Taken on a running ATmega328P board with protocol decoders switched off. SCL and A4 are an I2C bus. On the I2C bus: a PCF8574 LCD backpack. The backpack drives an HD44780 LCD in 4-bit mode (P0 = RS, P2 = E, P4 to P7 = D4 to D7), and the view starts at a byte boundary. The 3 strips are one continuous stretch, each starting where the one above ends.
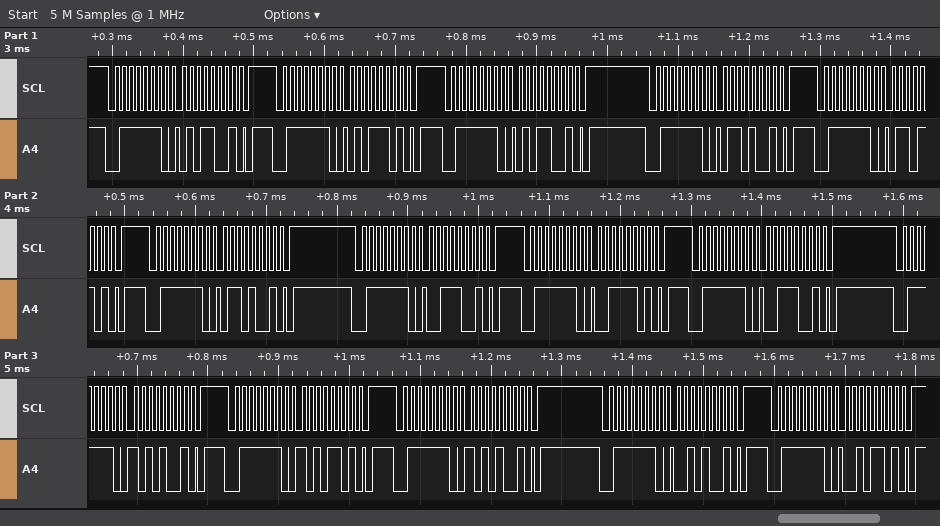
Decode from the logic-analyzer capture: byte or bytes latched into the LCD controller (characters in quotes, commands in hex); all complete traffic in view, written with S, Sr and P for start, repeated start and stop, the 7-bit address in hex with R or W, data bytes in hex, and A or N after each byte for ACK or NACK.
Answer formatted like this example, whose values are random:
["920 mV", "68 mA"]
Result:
["'V' ':'", "S 3FW A 59 A P S 3FW A 5D A P S 3FW A 59 A P S 3FW A 69 A P S 3FW A 6D A P S 3FW A 69 A P S 3FW A 39 A P S 3FW A 3D A P S 3FW A 39 A P S 3FW A A9 A P S 3FW A AD A P S 3FW A A9 A P S 3FW A 29 A P S 3FW A 2D A P"]
